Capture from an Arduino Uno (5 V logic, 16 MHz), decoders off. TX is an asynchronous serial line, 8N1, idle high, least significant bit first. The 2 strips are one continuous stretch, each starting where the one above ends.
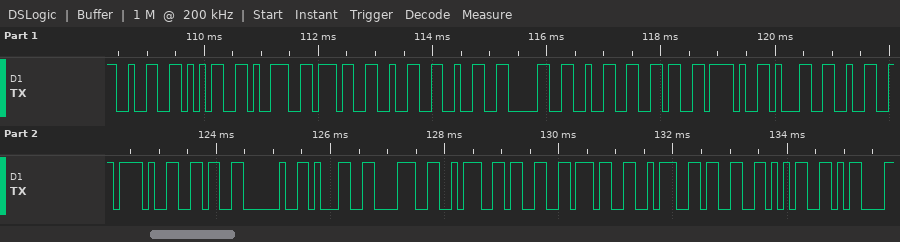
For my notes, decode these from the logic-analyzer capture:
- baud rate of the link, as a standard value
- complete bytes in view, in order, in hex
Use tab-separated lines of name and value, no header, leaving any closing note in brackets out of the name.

baud rate of the link, as a standard value	9600 baud
complete bytes in view, in order, in hex	0x32 0x35 0x39 0x37 0x32 0x32 0x30 0x32 0x36 0x2F 0x31 0x32 0x2F 0x36 0x20 0x31 0x38 0x3A 0x33 0x37 0x3A 0x33 0x35 0x0D
